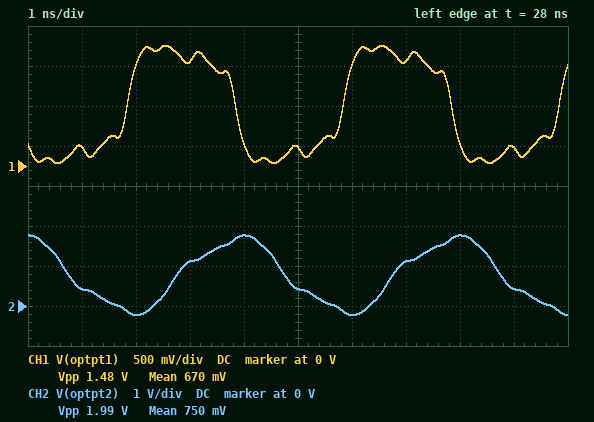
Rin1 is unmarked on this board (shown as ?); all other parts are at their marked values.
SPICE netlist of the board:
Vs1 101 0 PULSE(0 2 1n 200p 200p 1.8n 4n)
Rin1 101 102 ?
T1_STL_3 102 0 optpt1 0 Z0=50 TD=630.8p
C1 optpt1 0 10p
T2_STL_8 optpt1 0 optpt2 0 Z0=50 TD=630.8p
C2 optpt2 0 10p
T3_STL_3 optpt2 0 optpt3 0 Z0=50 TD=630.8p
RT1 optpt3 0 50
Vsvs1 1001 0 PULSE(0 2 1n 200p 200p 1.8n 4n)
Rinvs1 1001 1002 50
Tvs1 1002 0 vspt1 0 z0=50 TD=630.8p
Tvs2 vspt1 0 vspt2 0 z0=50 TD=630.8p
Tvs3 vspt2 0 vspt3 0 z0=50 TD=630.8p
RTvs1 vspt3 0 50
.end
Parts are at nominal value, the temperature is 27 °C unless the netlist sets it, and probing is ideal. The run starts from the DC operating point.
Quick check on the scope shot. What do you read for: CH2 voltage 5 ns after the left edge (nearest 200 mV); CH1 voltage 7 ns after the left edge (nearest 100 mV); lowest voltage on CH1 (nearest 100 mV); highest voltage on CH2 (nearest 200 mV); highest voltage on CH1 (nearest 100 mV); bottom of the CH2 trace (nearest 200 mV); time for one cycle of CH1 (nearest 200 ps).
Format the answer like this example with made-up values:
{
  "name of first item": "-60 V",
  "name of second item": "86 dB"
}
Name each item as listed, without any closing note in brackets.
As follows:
{
  "CH2 voltage 5 ns after the left edge": "400 mV",
  "CH1 voltage 7 ns after the left edge": "1.3 V",
  "lowest voltage on CH1": "0 V",
  "highest voltage on CH2": "1.8 V",
  "highest voltage on CH1": "1.5 V",
  "bottom of the CH2 trace": "-200 mV",
  "time for one cycle of CH1": "4.0 ns"
}
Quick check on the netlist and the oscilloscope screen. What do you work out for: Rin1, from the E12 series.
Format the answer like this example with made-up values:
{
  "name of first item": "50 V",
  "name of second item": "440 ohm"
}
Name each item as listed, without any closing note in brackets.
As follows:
{
  "Rin1, from the E12 series": "15 Ω"
}
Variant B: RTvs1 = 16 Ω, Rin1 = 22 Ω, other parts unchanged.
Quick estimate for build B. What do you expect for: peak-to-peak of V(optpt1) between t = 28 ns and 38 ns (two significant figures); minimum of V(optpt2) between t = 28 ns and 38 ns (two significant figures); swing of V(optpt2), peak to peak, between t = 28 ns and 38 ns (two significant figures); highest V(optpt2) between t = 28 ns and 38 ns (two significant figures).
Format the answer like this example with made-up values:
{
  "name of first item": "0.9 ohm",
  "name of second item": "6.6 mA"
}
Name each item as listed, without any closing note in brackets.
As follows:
{
  "peak-to-peak of V(optpt1) between t = 28 ns and 38 ns": "1.4 V",
  "minimum of V(optpt2) between t = 28 ns and 38 ns": "-190 mV",
  "swing of V(optpt2), peak to peak, between t = 28 ns and 38 ns": "1.8 V",
  "highest V(optpt2) between t = 28 ns and 38 ns": "1.6 V"
}
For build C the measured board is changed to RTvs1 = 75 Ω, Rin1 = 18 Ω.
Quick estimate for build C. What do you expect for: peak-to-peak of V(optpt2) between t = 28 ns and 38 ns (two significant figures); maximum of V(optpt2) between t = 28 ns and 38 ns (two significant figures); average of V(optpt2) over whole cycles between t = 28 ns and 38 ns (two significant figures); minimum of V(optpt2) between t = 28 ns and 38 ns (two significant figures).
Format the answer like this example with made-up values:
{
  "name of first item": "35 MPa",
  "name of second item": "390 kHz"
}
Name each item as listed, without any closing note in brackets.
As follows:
{
  "peak-to-peak of V(optpt2) between t = 28 ns and 38 ns": "1.9 V",
  "maximum of V(optpt2) between t = 28 ns and 38 ns": "1.7 V",
  "average of V(optpt2) over whole cycles between t = 28 ns and 38 ns": "740 mV",
  "minimum of V(optpt2) between t = 28 ns and 38 ns": "-210 mV"
}
